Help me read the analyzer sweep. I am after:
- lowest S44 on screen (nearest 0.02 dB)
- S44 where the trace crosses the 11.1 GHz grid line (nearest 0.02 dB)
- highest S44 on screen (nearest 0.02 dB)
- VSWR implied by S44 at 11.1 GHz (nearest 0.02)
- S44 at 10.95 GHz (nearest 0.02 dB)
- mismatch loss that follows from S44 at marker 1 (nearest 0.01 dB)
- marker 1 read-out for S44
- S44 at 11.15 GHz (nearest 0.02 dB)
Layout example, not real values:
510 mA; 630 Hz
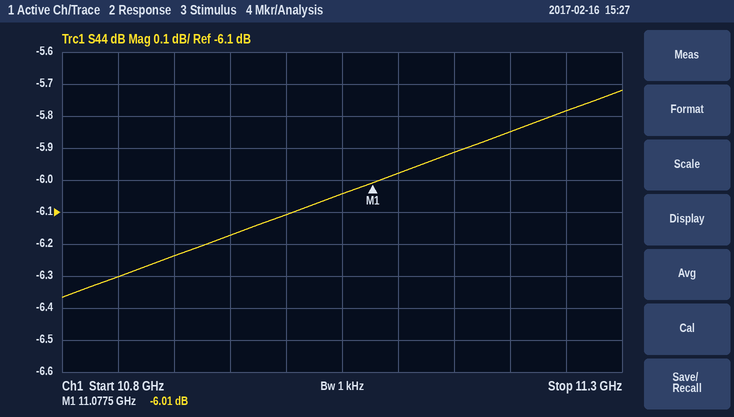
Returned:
-6.36 dB; -5.98 dB; -5.72 dB; 3.02; -6.18 dB; 1.25 dB; -6.01 dB; -5.92 dB
